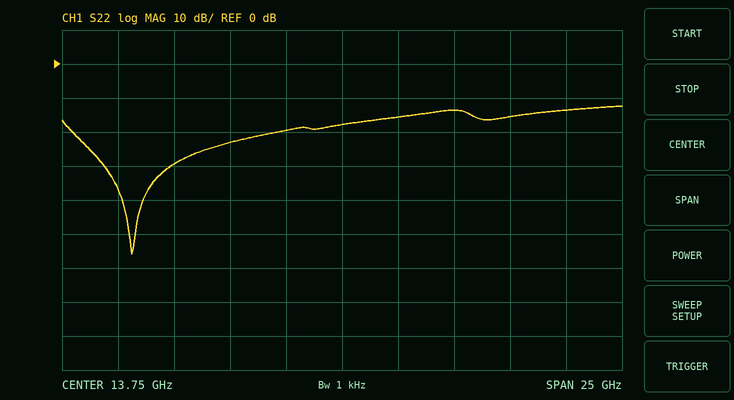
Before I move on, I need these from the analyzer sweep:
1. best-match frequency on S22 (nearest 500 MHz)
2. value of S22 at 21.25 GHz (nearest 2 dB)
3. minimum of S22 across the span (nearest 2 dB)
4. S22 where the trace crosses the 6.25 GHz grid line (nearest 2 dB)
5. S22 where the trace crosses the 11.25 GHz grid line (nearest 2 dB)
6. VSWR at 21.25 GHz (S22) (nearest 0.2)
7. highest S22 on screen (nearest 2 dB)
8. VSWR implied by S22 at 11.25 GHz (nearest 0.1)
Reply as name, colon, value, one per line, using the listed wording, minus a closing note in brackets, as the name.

best-match frequency on S22: 4.5 GHz
value of S22 at 21.25 GHz: -16 dB
minimum of S22 across the span: -56 dB
S22 where the trace crosses the 6.25 GHz grid line: -30 dB
S22 where the trace crosses the 11.25 GHz grid line: -20 dB
VSWR at 21.25 GHz (S22): 1.4
highest S22 on screen: -12 dB
VSWR implied by S22 at 11.25 GHz: 1.2
